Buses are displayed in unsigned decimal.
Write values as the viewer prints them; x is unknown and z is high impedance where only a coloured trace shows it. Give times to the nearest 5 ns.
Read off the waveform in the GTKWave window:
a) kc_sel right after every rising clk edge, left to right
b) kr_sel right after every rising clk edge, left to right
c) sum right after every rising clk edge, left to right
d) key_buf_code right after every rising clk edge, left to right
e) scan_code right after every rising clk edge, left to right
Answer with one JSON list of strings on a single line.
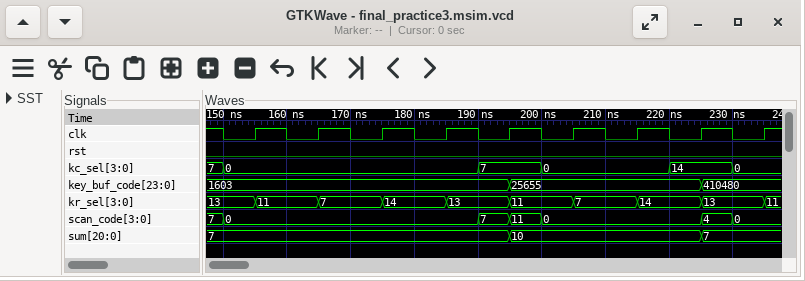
["0, 0, 0, 0, 7, 0, 0, 14, 0", "11, 7, 14, 13, 11, 7, 14, 13, 11", "7, 7, 7, 7, 10, 10, 10, 7, 7", "1603, 1603, 1603, 1603, 25655, 25655, 25655, 410480, 410480", "0, 0, 0, 0, 11, 0, 0, 4, 0"]
